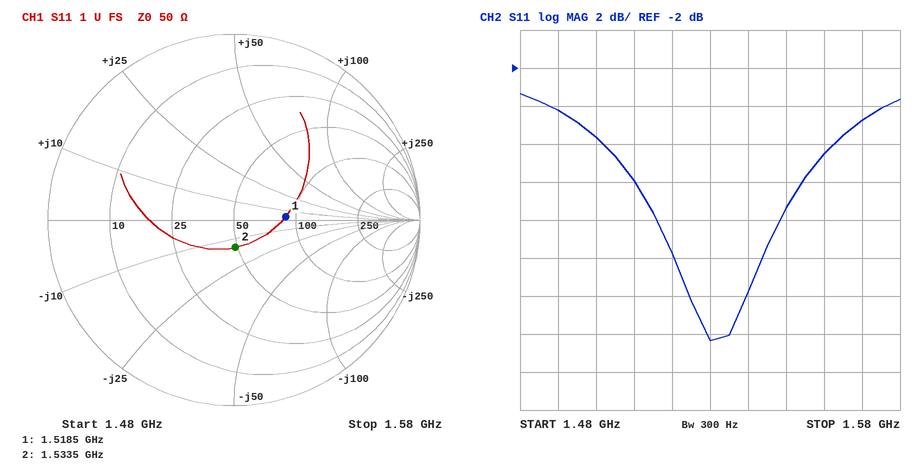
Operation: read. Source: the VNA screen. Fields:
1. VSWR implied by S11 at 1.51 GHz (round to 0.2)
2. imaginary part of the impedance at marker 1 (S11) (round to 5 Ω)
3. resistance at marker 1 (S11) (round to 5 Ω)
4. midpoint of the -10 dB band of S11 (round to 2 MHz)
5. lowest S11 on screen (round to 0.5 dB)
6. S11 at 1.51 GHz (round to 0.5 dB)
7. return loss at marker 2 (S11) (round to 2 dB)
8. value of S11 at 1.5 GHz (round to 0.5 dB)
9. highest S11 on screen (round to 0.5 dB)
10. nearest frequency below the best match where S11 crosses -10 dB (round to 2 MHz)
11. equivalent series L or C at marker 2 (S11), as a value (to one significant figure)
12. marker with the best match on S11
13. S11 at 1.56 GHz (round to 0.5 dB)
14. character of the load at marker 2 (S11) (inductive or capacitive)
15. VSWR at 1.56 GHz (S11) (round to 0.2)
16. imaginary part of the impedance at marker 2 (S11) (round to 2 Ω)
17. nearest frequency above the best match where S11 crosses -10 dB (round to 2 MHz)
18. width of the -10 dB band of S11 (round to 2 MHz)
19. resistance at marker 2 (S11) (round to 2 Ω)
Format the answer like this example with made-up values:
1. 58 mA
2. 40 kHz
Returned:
1. 2.4
2. +5 Ω
3. 90 Ω
4. 1.532 GHz
5. -16.5 dB
6. -8.0 dB
7. 16 dB
8. -5.5 dB
9. -3.5 dB
10. 1.516 GHz
11. 7 pF
12. marker 2
13. -6.5 dB
14. capacitive
15. 2.8
16. -14 Ω
17. 1.548 GHz
18. 32 MHz
19. 48 Ω
